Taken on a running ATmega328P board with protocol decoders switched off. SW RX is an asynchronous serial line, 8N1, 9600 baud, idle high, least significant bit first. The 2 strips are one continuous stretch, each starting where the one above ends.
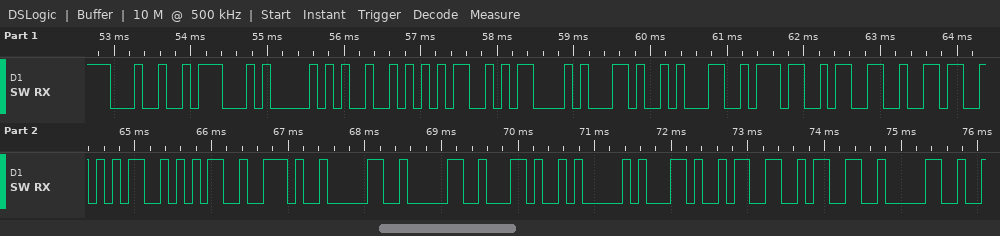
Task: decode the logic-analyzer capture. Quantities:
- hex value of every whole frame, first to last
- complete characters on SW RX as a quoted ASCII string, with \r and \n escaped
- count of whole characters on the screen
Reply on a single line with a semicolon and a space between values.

24 47 50 52 4D 43 2C 31 37 33 36 35 35 2E 30 30 2C 41 2C 33 33 30; "$GPRMC,173655.00,A,330"; 22
